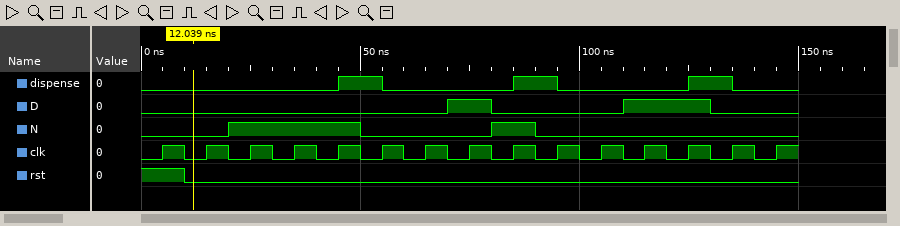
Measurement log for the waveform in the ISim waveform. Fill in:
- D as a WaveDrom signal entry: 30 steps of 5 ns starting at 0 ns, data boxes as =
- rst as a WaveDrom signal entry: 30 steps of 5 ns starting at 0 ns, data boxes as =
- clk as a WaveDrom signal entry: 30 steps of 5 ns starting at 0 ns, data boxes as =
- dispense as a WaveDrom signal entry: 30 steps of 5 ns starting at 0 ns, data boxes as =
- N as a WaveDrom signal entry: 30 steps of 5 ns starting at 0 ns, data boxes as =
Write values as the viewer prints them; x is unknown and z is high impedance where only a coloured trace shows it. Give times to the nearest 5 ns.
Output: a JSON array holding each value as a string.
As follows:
["{name: 'D', wave: '0.............1.0.....1...0...'}", "{name: 'rst', wave: '1.0...........................'}", "{name: 'clk', wave: '010101010101010101010101010101'}", "{name: 'dispense', wave: '0........1.0.....1.0.....1.0..'}", "{name: 'N', wave: '0...1.....0.....1.0...........'}"]
